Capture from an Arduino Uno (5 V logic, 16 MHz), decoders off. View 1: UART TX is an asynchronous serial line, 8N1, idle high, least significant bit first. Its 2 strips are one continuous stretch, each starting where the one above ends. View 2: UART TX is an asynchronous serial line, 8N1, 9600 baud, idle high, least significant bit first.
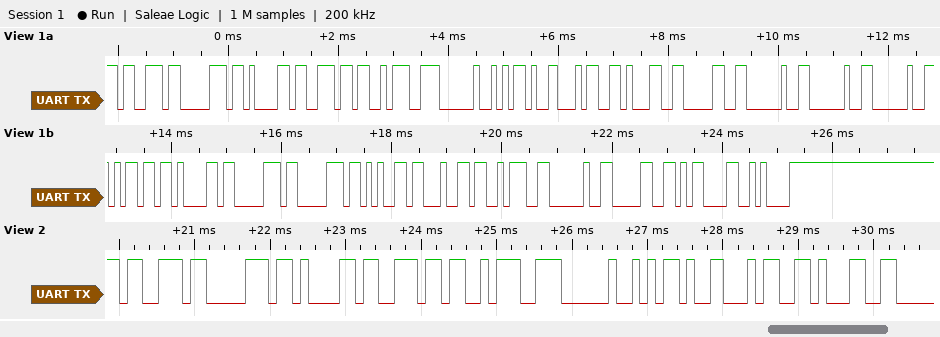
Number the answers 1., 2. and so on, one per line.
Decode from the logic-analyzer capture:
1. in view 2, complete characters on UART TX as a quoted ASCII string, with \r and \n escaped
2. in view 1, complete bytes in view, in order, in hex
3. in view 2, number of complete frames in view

1. "span: -41"
2. 0x73 0x70 0x61 0x6E 0x3A 0x20 0x2D 0x34 0x31 0x30 0x20 0x20 0x20 0x6D 0x61 0x70 0x70 0x65 0x64 0x3A 0x20 0x30 0x0D 0x0A
3. 9
